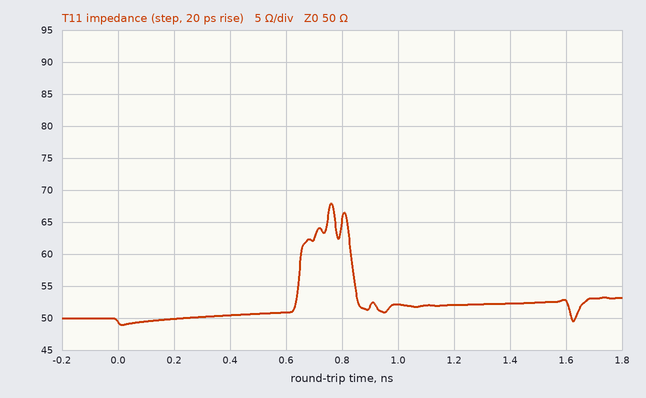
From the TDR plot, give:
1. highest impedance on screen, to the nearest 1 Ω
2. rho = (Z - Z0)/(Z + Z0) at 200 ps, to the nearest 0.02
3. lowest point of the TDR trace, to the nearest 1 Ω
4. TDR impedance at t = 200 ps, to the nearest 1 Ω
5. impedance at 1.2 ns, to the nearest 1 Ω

68 Ω
0.00
49 Ω
50 Ω
52 Ω
